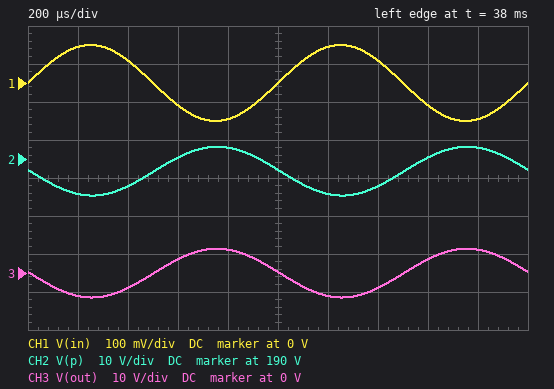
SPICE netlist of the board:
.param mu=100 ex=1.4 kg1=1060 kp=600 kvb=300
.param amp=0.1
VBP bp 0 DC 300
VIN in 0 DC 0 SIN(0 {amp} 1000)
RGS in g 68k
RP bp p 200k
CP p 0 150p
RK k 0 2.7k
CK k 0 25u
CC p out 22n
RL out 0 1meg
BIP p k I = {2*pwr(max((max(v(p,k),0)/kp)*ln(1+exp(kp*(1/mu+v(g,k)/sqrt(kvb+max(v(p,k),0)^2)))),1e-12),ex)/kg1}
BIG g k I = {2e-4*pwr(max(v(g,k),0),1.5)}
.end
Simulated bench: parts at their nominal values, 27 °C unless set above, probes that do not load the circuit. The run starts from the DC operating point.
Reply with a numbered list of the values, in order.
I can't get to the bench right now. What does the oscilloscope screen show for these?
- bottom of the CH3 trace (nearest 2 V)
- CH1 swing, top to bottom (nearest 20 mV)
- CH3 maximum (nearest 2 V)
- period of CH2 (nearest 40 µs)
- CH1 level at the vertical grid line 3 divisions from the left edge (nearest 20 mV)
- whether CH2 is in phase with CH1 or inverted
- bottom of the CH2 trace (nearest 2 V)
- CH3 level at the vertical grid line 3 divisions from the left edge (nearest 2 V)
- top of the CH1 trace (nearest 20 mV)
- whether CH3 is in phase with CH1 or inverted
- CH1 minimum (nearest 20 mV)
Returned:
1. -6 V
2. 200 mV
3. 6 V
4. 1.00 ms
5. -60 mV
6. inverted
7. 180 V
8. 4 V
9. 100 mV
10. inverted
11. -100 mV
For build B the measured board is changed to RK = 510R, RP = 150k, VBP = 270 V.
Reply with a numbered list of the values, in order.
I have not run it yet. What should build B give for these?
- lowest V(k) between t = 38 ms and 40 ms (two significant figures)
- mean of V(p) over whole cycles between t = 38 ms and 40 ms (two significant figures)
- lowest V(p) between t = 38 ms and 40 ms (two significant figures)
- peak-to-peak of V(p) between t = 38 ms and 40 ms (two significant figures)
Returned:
1. 520 mV
2. 120 V
3. 110 V
4. 14 V
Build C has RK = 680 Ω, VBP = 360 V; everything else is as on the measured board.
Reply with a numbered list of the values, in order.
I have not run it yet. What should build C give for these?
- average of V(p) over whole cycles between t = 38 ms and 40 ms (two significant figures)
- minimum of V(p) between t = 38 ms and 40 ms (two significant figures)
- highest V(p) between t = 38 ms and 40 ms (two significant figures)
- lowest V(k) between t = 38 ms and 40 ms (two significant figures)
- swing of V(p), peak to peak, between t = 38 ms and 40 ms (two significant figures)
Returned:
1. 140 V
2. 130 V
3. 150 V
4. 740 mV
5. 15 V
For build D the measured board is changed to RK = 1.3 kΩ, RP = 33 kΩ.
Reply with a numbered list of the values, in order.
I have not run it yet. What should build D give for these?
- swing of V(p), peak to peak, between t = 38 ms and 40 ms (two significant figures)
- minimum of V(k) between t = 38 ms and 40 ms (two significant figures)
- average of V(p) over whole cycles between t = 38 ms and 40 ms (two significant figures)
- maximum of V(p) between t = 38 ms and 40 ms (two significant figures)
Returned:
1. 7.7 V
2. 1.8 V
3. 250 V
4. 260 V
